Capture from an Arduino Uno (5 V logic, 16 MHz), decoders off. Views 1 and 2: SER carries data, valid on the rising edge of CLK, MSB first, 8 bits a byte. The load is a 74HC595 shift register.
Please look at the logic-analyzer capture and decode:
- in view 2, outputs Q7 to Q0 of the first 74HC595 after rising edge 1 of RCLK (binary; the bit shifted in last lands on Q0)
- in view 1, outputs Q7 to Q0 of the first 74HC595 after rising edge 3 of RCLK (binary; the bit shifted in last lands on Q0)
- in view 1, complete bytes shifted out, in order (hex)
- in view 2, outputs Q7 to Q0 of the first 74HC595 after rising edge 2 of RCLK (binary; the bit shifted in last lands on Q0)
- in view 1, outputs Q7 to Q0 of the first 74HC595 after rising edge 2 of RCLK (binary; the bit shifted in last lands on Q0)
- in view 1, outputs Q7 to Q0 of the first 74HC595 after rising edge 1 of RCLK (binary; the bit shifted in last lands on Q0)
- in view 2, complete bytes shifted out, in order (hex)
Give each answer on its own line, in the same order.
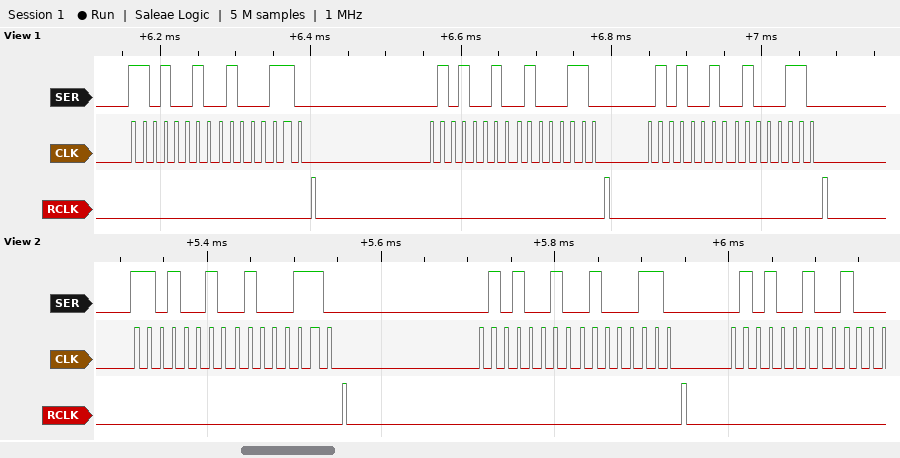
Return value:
01000110
01000110
D2 46 52 46 52 46
01000110
01000110
01000110
D2 46 52 46 52
